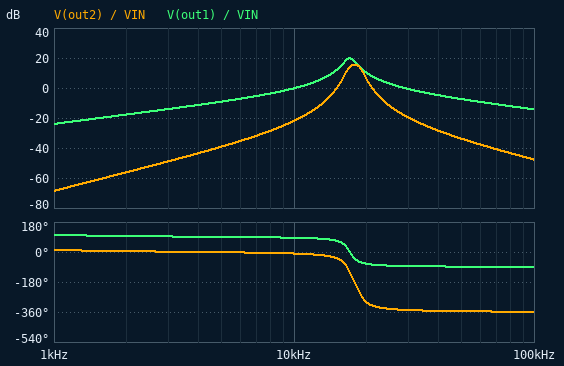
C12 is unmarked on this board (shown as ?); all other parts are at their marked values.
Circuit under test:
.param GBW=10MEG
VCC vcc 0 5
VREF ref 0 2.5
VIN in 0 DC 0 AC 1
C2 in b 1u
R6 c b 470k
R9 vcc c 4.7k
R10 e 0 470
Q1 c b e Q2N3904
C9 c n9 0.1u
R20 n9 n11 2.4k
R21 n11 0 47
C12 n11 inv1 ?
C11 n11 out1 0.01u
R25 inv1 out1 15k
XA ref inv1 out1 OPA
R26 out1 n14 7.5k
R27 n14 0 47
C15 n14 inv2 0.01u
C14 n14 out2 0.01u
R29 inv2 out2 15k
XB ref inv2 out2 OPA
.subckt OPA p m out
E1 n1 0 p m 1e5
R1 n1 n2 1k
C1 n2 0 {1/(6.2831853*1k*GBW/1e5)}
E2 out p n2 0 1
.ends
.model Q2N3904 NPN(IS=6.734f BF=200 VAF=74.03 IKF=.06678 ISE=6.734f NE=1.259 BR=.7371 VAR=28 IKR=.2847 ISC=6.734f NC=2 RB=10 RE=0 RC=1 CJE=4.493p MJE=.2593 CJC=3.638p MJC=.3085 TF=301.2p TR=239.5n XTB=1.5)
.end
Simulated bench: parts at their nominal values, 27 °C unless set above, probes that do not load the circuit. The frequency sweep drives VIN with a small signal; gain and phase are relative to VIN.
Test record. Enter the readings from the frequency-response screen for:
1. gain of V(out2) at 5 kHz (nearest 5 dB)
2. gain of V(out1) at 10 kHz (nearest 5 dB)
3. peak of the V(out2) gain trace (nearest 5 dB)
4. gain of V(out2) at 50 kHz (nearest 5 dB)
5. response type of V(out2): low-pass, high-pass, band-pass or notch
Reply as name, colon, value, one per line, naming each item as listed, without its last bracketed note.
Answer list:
gain of V(out2) at 5 kHz: -40 dB
gain of V(out1) at 10 kHz: 0 dB
peak of the V(out2) gain trace: 15 dB
gain of V(out2) at 50 kHz: -35 dB
response type of V(out2): low-pass, high-pass, band-pass or notch: band-pass
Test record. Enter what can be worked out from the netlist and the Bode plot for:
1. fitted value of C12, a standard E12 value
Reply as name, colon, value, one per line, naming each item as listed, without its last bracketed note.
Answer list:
fitted value of C12, a standard E12 value: 12 nF
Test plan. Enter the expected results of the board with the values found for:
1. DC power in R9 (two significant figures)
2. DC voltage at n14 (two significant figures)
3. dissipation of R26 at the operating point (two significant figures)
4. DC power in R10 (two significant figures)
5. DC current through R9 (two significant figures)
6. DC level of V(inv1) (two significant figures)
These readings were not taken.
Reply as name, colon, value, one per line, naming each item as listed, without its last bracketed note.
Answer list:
DC power in R9: 840 µW
DC voltage at n14: 16 mV
dissipation of R26 at the operating point: 820 µW
DC power in R10: 84 µW
DC current through R9: 420 µA
DC level of V(inv1): 2.5 V
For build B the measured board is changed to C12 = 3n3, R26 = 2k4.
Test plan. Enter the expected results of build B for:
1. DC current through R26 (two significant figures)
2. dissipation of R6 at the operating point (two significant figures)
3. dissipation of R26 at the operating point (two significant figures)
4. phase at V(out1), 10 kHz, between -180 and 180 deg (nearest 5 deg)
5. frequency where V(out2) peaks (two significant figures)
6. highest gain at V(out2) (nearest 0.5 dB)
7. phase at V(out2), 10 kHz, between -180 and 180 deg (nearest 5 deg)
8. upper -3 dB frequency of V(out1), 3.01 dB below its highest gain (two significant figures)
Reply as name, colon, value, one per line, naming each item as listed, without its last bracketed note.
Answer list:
DC current through R26: 1.0 mA
dissipation of R6 at the operating point: 10 µW
dissipation of R26 at the operating point: 2.5 mW
phase at V(out1), 10 kHz, between -180 and 180 deg: 90 deg
frequency where V(out2) peaks: 19 kHz
highest gain at V(out2): 4.0 dB
phase at V(out2), 10 kHz, between -180 and 180 deg: -5 deg
upper -3 dB frequency of V(out1), 3.01 dB below its highest gain: 35 kHz
